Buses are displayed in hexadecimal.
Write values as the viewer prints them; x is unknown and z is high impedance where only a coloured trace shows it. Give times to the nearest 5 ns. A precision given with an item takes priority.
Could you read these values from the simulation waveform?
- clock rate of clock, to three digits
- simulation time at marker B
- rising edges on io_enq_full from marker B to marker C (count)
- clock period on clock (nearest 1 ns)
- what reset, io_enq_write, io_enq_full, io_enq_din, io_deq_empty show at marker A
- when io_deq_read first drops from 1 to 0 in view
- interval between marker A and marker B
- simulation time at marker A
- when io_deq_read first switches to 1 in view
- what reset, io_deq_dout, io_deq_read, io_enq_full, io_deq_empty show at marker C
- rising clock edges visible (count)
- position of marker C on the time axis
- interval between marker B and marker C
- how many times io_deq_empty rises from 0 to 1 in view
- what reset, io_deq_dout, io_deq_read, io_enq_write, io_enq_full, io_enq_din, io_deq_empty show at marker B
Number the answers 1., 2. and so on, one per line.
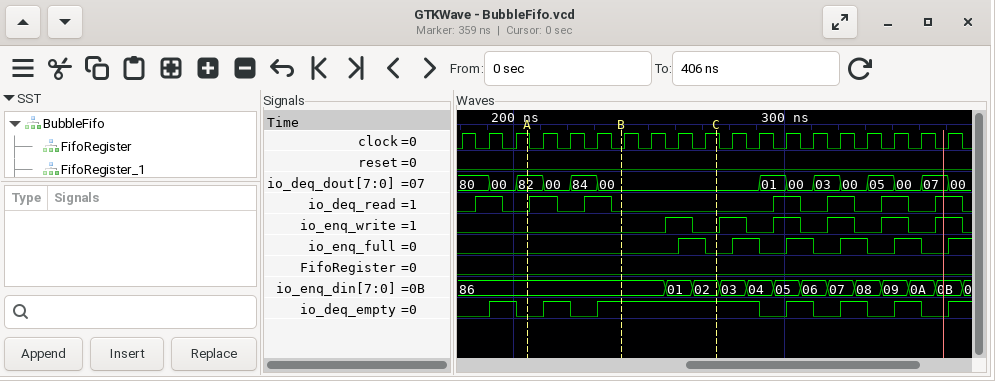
1. 100 MHz
2. 240 ns
3. 1
4. 10 ns
5. reset=0, io_enq_write=0, io_enq_full=0, io_enq_din=86, io_deq_empty=0
6. 195 ns
7. 35 ns
8. 205 ns
9. 185 ns
10. reset=0, io_deq_dout=00, io_deq_read=0, io_enq_full=0, io_deq_empty=1
11. 19
12. 275 ns
13. 35 ns
14. 7
15. reset=0, io_deq_dout=00, io_deq_read=0, io_enq_write=0, io_enq_full=0, io_enq_din=86, io_deq_empty=1
